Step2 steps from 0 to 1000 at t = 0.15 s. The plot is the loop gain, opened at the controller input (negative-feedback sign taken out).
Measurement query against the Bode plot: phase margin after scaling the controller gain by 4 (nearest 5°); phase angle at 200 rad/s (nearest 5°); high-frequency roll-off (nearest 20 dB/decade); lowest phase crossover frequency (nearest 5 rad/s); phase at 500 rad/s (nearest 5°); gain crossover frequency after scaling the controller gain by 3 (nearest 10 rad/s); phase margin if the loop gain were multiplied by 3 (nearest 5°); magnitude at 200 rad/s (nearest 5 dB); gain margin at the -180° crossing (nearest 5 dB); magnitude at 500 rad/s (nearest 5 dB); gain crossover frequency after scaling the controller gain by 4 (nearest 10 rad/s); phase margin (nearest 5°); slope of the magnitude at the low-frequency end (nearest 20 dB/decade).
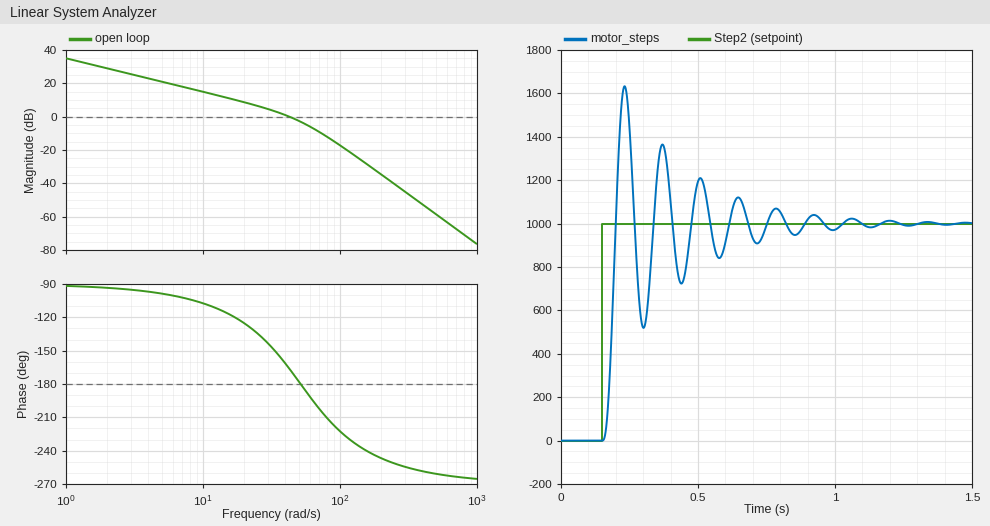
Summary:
-30°
-245°
-60 dB/decade
50 rad/s
-260°
70 rad/s
-25°
-35 dB
5 dB
-60 dB
80 rad/s
15°
-20 dB/decade
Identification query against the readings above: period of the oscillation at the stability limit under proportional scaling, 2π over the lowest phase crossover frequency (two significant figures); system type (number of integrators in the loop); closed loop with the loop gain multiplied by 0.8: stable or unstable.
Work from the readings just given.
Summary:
0.13 s
1
stable
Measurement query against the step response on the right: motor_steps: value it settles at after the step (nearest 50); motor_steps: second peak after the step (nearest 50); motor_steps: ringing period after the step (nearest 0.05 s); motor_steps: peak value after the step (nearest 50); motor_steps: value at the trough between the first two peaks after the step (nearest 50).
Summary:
1000
1350
0.15 s
1650
500
